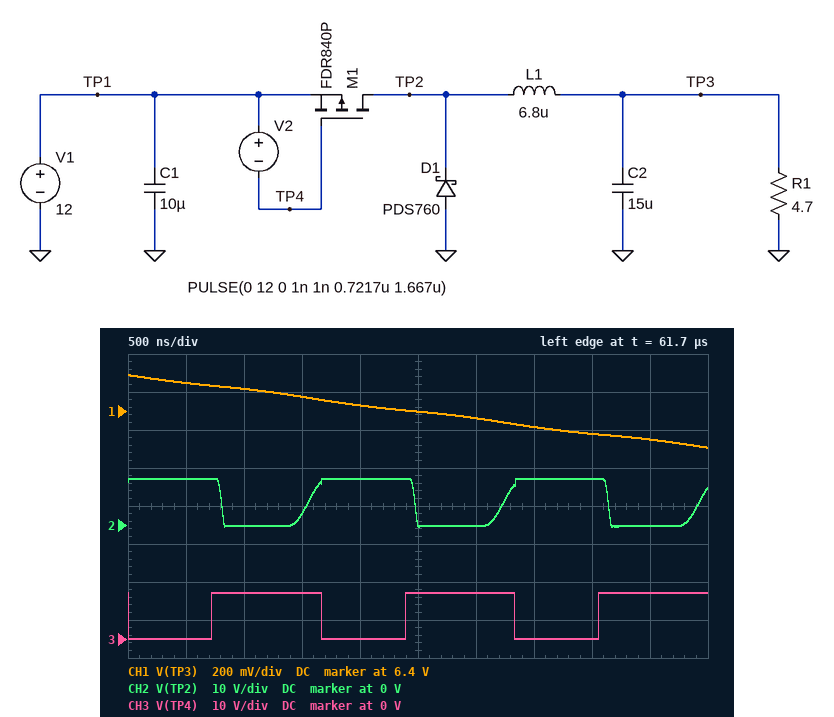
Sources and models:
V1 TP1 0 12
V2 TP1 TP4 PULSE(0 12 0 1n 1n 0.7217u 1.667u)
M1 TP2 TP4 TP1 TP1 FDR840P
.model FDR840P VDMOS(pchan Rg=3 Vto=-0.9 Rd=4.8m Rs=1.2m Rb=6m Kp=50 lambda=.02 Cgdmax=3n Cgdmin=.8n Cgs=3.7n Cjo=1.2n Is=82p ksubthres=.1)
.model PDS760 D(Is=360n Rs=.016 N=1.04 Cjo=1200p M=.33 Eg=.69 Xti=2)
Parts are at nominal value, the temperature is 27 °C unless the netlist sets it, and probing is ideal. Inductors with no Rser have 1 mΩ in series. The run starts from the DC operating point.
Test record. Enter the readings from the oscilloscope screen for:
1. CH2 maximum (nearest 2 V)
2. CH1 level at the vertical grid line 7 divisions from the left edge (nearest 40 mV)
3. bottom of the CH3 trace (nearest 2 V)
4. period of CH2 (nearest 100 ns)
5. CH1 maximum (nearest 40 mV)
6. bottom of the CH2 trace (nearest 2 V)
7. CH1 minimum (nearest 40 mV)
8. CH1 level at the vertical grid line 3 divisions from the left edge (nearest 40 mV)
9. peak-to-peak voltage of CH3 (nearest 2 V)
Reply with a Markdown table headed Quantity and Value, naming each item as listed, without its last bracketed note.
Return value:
| Quantity | Value |
|---|---|
| CH2 maximum | 12 V |
| CH1 level at the vertical grid line 7 divisions from the left edge | 6.32 V |
| bottom of the CH3 trace | 0 V |
| period of CH2 | 1.7 µs |
| CH1 maximum | 6.60 V |
| bottom of the CH2 trace | 0 V |
| CH1 minimum | 6.20 V |
| CH1 level at the vertical grid line 3 divisions from the left edge | 6.48 V |
| peak-to-peak voltage of CH3 | 12 V |
